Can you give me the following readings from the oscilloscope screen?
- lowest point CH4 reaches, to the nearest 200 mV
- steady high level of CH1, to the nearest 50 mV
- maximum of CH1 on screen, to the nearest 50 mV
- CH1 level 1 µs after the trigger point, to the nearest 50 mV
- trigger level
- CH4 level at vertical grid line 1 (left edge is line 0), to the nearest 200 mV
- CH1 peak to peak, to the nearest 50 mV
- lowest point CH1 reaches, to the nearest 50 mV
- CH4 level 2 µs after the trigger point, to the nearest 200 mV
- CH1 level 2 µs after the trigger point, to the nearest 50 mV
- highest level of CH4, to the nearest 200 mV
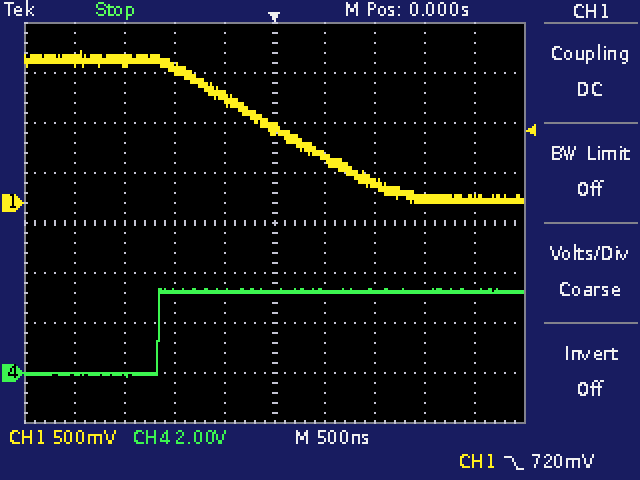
-200 mV
1.45 V
1.50 V
200 mV
720 mV
0.0 V
1.50 V
0 mV
3.2 V
50 mV
3.4 V
